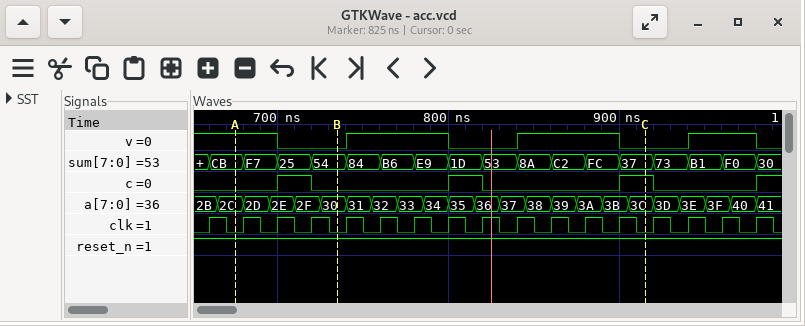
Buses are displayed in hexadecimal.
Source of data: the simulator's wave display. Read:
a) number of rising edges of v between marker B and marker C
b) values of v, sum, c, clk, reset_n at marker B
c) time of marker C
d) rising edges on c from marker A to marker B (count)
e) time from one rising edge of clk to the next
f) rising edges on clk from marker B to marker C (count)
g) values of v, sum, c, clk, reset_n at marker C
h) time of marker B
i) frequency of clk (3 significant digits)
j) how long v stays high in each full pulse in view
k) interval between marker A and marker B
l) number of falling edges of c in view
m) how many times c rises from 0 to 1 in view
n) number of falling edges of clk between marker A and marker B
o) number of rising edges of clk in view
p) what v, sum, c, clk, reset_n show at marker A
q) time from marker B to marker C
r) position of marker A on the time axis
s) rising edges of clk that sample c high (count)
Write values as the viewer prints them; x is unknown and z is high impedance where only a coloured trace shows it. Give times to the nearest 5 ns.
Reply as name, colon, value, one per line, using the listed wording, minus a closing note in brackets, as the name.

number of rising edges of v between marker B and marker C: 2
values of v, sum, c, clk, reset_n at marker B: v=0, sum=54, c=0, clk=0, reset_n=1
time of marker C: 915 ns
rising edges on c from marker A to marker B: 1
time from one rising edge of clk to the next: 20 ns
rising edges on clk from marker B to marker C: 9
values of v, sum, c, clk, reset_n at marker C: v=0, sum=37, c=1, clk=0, reset_n=1
time of marker B: 735 ns
frequency of clk: 50.0 MHz
how long v stays high in each full pulse in view: 60 ns, 60 ns, 40 ns
interval between marker A and marker B: 60 ns
number of falling edges of c in view: 3
how many times c rises from 0 to 1 in view: 4
number of falling edges of clk between marker A and marker B: 3
number of rising edges of clk in view: 17
what v, sum, c, clk, reset_n show at marker A: v=1, sum=CB, c=0, clk=0, reset_n=1
time from marker B to marker C: 180 ns
position of marker A on the time axis: 675 ns
rising edges of clk that sample c high: 3
